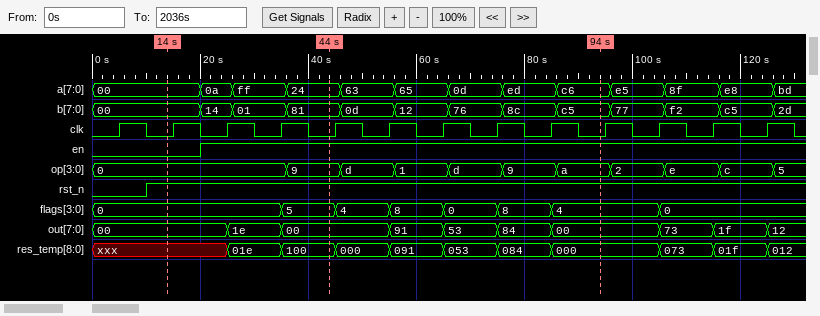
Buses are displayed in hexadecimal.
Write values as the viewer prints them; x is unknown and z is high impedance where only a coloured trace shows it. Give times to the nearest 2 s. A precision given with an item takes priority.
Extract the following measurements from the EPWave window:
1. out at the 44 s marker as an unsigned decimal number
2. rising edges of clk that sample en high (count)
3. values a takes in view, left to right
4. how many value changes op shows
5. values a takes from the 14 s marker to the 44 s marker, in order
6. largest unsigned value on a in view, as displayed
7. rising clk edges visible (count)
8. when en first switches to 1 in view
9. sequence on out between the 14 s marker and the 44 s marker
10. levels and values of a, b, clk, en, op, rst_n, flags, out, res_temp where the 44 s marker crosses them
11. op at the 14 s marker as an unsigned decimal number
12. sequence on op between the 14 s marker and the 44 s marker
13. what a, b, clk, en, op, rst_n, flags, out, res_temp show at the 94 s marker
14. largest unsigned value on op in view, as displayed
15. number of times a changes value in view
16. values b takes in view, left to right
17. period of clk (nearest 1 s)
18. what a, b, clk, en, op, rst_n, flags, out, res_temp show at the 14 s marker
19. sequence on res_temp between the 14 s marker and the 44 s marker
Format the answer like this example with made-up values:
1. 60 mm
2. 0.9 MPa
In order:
1. 0
2. 11
3. 00, 0a, ff, 24, 63, 65, 0d, ed, c6, e5, 8f, e8, bd
4. 10
5. 00, 0a, ff, 24
6. ff
7. 13
8. 20 s
9. 00, 1e, 00
10. a=24, b=81, clk=0, en=1, op=9, rst_n=1, flags=5, out=00, res_temp=100
11. 0
12. 0, 9
13. a=c6, b=c5, clk=0, en=1, op=a, rst_n=1, flags=4, out=00, res_temp=000
14. e
15. 12
16. 00, 14, 01, 81, 0d, 12, 76, 8c, c5, 77, f2, c5, 2d
17. 10 s
18. a=00, b=00, clk=0, en=0, op=0, rst_n=1, flags=0, out=00, res_temp=xxx
19. xxx, 01e, 100
